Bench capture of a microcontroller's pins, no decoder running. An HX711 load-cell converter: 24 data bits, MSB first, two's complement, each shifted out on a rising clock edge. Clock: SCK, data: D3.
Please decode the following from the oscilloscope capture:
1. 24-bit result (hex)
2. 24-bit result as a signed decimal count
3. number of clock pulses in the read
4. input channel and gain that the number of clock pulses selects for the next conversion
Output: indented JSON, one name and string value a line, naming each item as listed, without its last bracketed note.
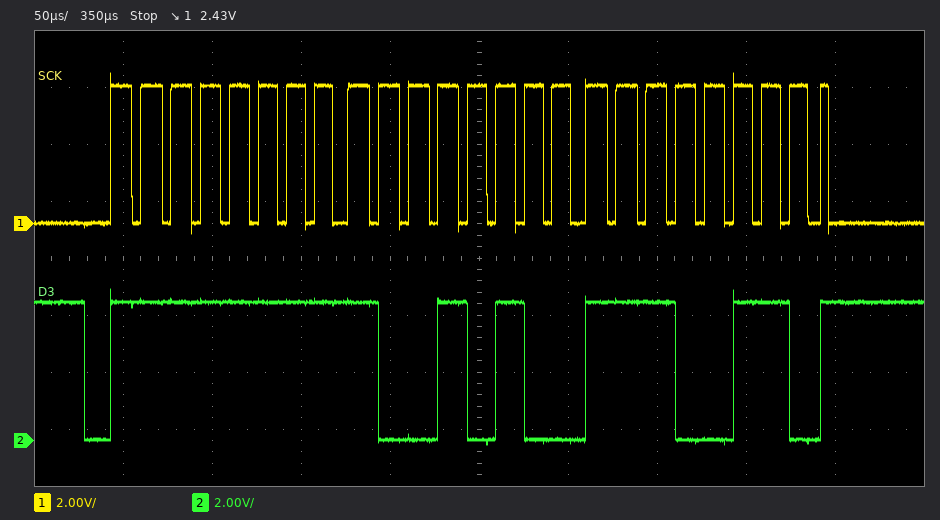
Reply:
{
  "24-bit result": "0xFF94E6",
  "24-bit result as a signed decimal count": "-27418",
  "number of clock pulses in the read": "25",
  "input channel and gain that the number of clock pulses selects for the next conversion": "channel A, gain 128"
}
